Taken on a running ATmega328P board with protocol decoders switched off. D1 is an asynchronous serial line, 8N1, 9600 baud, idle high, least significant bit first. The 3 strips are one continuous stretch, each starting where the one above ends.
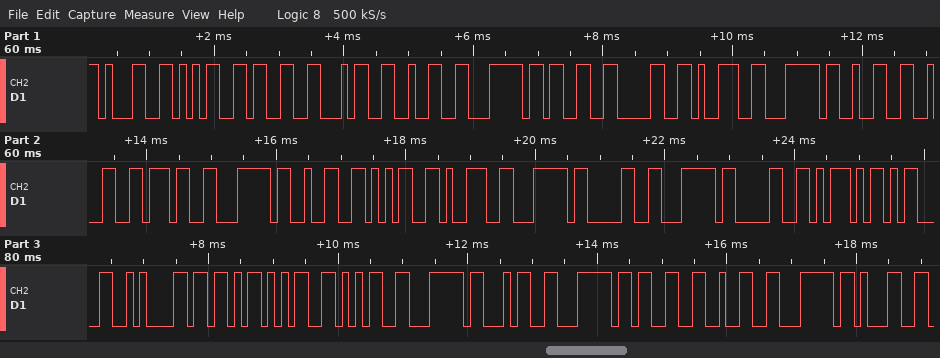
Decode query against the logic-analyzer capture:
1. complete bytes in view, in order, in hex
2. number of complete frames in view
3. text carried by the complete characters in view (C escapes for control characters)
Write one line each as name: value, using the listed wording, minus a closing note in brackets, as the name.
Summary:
complete bytes in view, in order, in hex: 0x31 0x35 0x33 0x34 0x32 0x7C 0x33 0x30 0x39 0x7C 0x32 0x32 0x37 0x7C 0x32 0x35 0x39 0x7C 0x30 0x7C 0x30 0x5D 0x0D 0x0A 0x5B 0x35 0x35 0x7C 0x34 0x7C 0x33 0x32 0x7C 0x31
number of complete frames in view: 34
text carried by the complete characters in view: "15342|309|227|259|0|0]\r\n[55|4|32|1"
